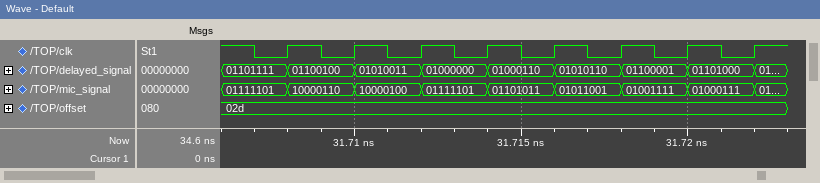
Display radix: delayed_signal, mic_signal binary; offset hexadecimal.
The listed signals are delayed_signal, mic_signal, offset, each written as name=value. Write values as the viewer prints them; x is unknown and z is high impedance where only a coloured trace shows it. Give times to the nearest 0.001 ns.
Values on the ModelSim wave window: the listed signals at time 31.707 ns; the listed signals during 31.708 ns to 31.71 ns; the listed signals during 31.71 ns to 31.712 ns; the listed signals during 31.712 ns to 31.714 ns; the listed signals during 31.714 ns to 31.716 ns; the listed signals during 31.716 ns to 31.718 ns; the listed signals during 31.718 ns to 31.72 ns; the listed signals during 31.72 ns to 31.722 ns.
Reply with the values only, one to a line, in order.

delayed_signal=01101111, mic_signal=01111101, offset=02d
delayed_signal=01100100, mic_signal=10000110, offset=02d
delayed_signal=01010011, mic_signal=10000100, offset=02d
delayed_signal=01000000, mic_signal=01111101, offset=02d
delayed_signal=01000110, mic_signal=01101011, offset=02d
delayed_signal=01010110, mic_signal=01011001, offset=02d
delayed_signal=01100001, mic_signal=01001111, offset=02d
delayed_signal=01101000, mic_signal=01000111, offset=02d
